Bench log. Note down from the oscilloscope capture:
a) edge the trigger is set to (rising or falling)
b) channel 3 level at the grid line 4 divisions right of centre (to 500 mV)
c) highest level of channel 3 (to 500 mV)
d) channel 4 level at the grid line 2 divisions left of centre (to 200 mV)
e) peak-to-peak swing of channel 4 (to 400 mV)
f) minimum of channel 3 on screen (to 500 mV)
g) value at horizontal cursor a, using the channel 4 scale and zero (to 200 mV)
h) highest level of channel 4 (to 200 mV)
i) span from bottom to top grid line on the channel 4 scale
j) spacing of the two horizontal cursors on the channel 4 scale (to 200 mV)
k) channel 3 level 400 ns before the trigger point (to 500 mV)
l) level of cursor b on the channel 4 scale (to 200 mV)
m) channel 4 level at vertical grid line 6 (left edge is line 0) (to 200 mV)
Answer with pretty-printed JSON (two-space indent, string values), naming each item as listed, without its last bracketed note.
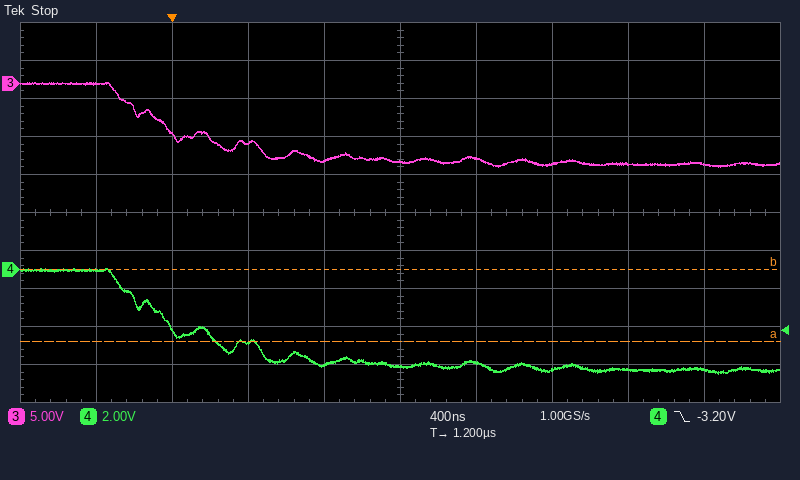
{
  "edge the trigger is set to": "falling",
  "channel 3 level at the grid line 4 divisions right of centre": "-10.5 V",
  "highest level of channel 3": "0.0 V",
  "channel 4 level at the grid line 2 divisions left of centre": "-3.8 V",
  "peak-to-peak swing of channel 4": "5.6 V",
  "minimum of channel 3 on screen": "-11.0 V",
  "value at horizontal cursor a, using the channel 4 scale and zero": "-3.8 V",
  "highest level of channel 4": "0.0 V",
  "span from bottom to top grid line on the channel 4 scale": "20 V",
  "spacing of the two horizontal cursors on the channel 4 scale": "3.8 V",
  "channel 3 level 400 ns before the trigger point": "0.0 V",
  "level of cursor b on the channel 4 scale": "0.0 V",
  "channel 4 level at vertical grid line 6 (left edge is line 0)": "-5.0 V"
}
